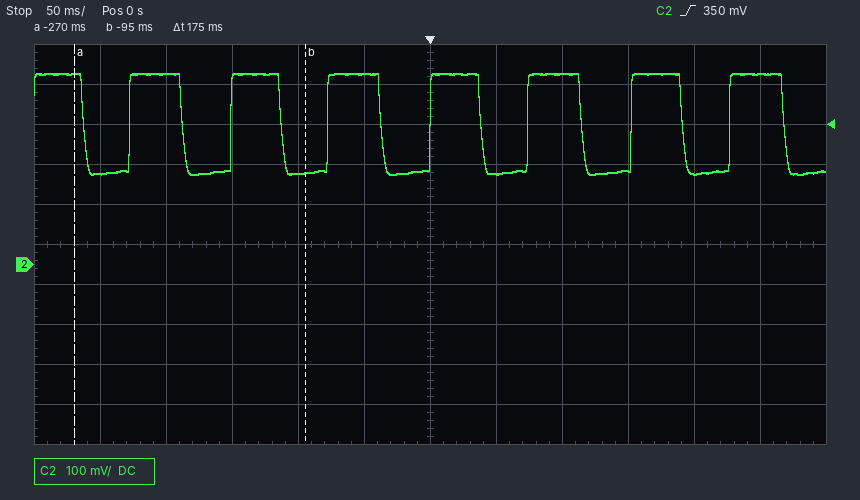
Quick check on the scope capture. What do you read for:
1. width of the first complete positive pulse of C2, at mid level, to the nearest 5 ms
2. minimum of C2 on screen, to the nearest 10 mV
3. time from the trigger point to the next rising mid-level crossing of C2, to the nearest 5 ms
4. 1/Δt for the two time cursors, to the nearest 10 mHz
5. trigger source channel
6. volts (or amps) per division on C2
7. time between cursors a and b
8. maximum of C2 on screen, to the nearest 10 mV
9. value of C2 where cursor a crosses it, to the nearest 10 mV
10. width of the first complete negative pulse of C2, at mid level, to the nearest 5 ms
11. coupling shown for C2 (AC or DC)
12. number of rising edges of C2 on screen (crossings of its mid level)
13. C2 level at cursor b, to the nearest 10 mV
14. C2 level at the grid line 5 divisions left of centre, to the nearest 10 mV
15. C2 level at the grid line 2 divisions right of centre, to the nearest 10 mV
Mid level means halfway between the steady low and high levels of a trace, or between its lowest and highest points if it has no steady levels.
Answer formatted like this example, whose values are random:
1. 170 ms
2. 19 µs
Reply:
1. 40 ms
2. 220 mV
3. 75 ms
4. 5.71 Hz
5. C2
6. 100 mV
7. 175 ms
8. 480 mV
9. 480 mV
10. 35 ms
11. DC
12. 7
13. 230 mV
14. 230 mV
15. 480 mV
